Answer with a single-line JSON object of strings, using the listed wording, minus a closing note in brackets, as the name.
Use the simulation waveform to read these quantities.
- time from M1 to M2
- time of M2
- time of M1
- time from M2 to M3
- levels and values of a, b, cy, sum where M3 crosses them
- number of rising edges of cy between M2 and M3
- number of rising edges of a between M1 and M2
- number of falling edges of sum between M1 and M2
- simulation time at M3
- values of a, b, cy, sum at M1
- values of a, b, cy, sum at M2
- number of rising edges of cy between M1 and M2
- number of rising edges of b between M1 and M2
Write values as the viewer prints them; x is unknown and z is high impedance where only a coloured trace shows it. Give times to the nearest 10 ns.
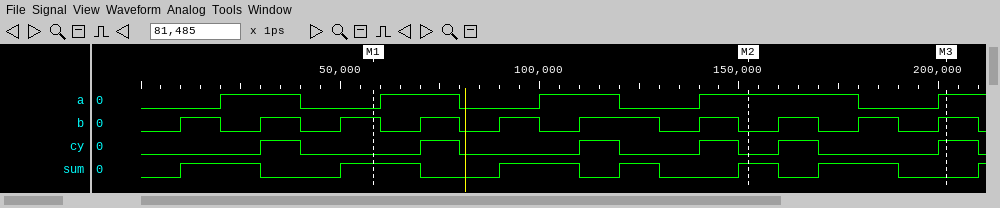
{"time from M1 to M2": "90 ns", "time of M2": "150 ns", "time of M1": "60 ns", "time from M2 to M3": "50 ns", "levels and values of a, b, cy, sum where M3 crosses them": "a=1, b=1, cy=1, sum=0", "number of rising edges of cy between M2 and M3": "2", "number of rising edges of a between M1 and M2": "3", "number of falling edges of sum between M1 and M2": "3", "simulation time at M3": "200 ns", "values of a, b, cy, sum at M1": "a=0, b=1, cy=0, sum=1", "values of a, b, cy, sum at M2": "a=1, b=0, cy=0, sum=1", "number of rising edges of cy between M1 and M2": "3", "number of rising edges of b between M1 and M2": "4"}
